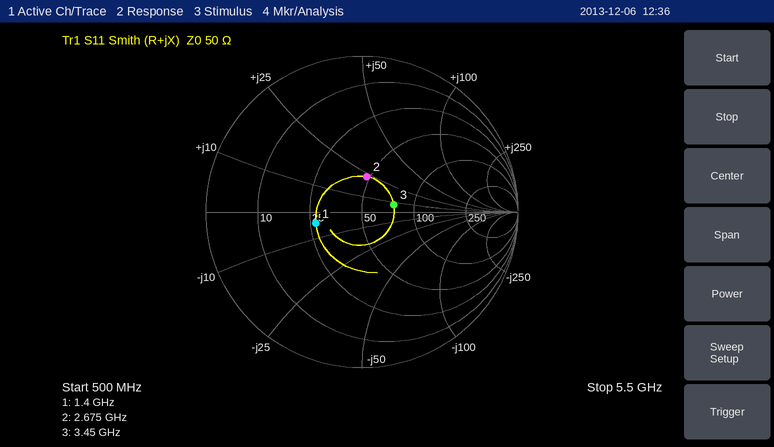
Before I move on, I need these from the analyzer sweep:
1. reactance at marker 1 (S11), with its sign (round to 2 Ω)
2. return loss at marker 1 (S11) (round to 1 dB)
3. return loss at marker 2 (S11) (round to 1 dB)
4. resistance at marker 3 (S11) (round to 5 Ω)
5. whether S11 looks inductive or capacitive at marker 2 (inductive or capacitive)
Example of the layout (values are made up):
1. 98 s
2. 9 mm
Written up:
1. -4 Ω
2. 10 dB
3. 13 dB
4. 75 Ω
5. inductive
